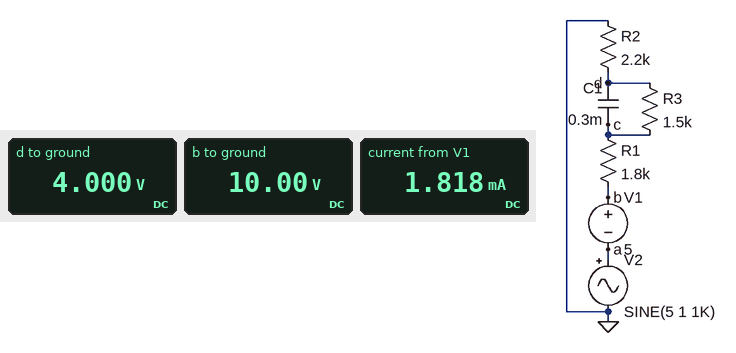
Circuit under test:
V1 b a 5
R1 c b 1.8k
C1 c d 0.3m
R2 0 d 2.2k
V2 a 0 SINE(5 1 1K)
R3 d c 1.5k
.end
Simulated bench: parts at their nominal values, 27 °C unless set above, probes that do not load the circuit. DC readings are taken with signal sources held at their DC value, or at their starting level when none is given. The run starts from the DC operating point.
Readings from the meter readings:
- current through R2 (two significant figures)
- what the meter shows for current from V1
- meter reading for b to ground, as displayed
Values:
1.8 mA
1.818 mA
10.00 V
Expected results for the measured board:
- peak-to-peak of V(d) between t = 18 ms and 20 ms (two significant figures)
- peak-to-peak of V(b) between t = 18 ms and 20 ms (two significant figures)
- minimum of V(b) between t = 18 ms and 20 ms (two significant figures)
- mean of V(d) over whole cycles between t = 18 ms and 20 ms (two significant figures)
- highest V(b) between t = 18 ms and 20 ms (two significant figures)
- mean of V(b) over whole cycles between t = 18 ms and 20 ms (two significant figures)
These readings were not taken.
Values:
1.1 V
2.0 V
9.0 V
4.0 V
11 V
10 V
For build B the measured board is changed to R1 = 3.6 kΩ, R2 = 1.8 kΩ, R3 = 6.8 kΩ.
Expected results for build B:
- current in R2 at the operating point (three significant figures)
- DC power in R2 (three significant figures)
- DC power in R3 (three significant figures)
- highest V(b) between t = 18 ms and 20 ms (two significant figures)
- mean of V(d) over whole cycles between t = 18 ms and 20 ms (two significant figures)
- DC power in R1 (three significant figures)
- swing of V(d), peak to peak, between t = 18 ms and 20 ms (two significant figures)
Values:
820 µA
1.21 mW
4.57 mW
11 V
1.5 V
2.42 mW
670 mV
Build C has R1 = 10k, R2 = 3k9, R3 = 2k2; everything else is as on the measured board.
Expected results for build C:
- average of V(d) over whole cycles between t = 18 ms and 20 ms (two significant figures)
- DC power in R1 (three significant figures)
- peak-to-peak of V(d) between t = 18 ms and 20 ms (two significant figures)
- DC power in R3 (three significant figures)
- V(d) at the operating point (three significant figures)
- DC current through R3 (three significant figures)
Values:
2.4 V
3.86 mW
560 mV
849 µW
2.42 V
621 µA
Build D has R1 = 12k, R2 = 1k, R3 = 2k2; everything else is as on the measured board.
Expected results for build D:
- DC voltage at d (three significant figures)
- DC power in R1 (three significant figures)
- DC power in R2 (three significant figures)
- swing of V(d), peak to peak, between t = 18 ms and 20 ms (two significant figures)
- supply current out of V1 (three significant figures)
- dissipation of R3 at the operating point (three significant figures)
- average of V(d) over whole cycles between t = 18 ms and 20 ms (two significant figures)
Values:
658 mV
5.19 mW
433 µW
150 mV
658 µA
952 µW
660 mV
